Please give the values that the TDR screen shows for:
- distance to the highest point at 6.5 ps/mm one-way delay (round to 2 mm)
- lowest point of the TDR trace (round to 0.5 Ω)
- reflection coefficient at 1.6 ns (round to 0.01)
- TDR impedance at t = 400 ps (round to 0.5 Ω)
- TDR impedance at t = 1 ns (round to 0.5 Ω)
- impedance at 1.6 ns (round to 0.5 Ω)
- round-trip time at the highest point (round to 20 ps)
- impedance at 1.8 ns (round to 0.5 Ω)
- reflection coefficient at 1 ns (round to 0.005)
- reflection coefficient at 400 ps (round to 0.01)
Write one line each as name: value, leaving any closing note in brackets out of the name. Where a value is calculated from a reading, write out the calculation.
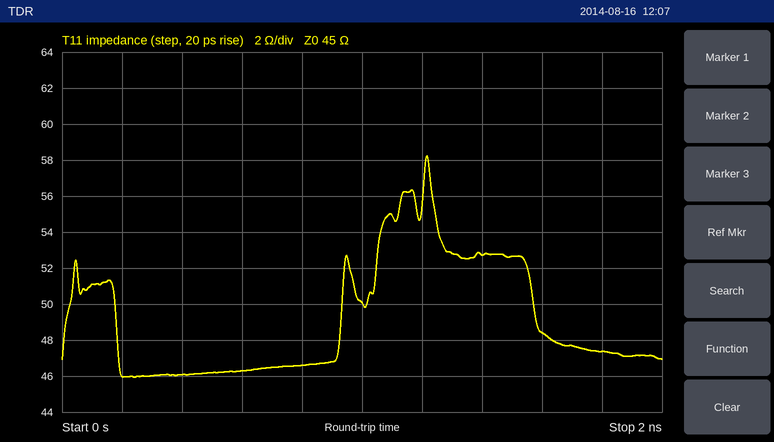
distance to the highest point at 6.5 ps/mm one-way delay: 1.22 ns / 2 / 6.5 ps/mm ≈ 94 mm
lowest point of the TDR trace: 46.0 Ω
reflection coefficient at 1.6 ns: (48.5 − 45)/(48.5 + 45) ≈ +0.04
TDR impedance at t = 400 ps: 46.0 Ω
TDR impedance at t = 1 ns: 50.0 Ω
impedance at 1.6 ns: 48.5 Ω
round-trip time at the highest point: 1.22 ns
impedance at 1.8 ns: 47.5 Ω
reflection coefficient at 1 ns: (50 − 45)/(50 + 45) ≈ +0.0526, so +0.055 to the nearest 0.005
reflection coefficient at 400 ps: (46 − 45)/(46 + 45) ≈ +0.01
